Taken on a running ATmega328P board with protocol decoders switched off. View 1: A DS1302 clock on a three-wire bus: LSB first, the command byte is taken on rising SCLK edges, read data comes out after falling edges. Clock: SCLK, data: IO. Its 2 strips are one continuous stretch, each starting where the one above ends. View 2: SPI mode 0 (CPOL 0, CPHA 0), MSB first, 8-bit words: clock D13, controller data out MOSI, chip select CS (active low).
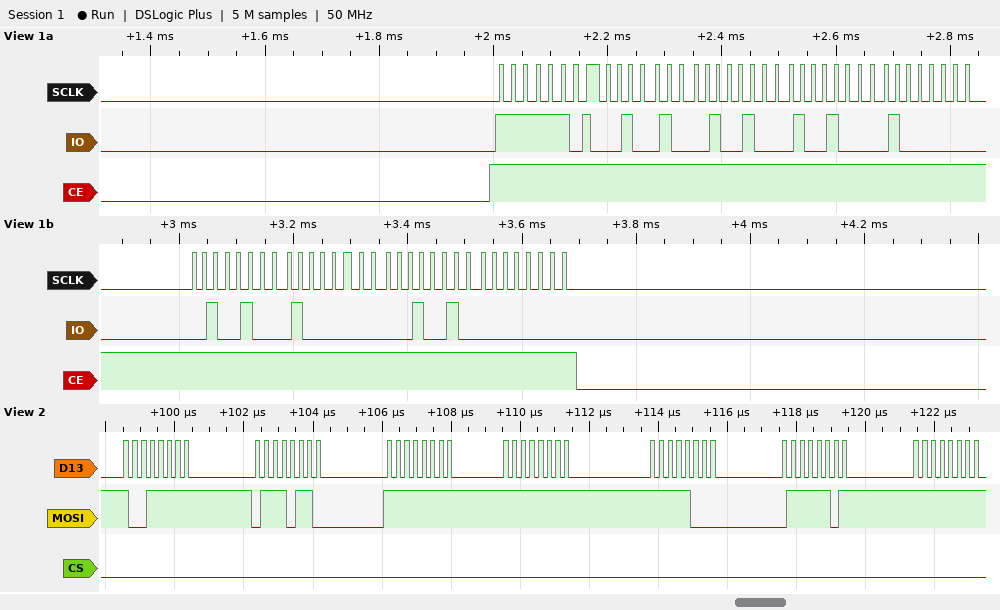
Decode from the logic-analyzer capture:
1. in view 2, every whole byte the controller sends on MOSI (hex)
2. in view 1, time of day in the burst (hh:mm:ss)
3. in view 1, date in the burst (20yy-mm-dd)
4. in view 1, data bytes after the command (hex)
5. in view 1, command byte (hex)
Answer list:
0x9F 0x76 0xFF 0xFF 0xF8 0x7D 0xFF
09:12:24
2024-12-01
24 12 09 01 12 01 24 00
0xBF
